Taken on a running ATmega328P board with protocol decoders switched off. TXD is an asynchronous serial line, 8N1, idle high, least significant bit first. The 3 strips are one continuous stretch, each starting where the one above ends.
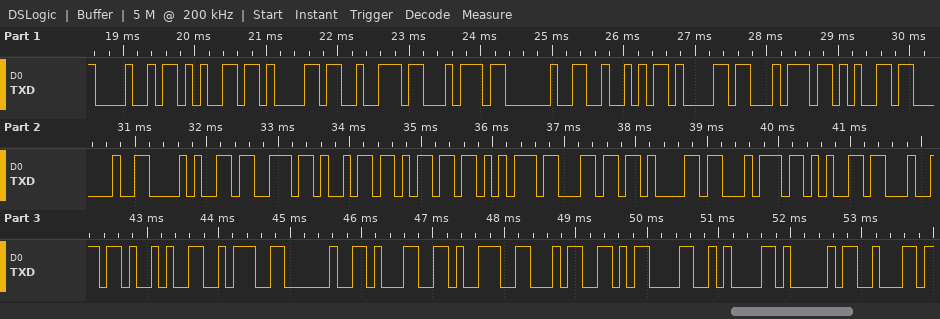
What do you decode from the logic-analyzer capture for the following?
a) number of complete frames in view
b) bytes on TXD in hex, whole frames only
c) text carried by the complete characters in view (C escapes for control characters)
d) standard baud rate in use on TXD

31
0x48 0x65 0x61 0x72 0x74 0x20 0x52 0x61 0x74 0x65 0x20 0x28 0x73 0x69 0x6D 0x75 0x6C 0x61 0x74 0x65 0x64 0x29 0x3A 0x20 0x31 0x39 0x34 0x0D 0x0A 0x41 0x62
"Heart Rate (simulated): 194\r\nAb"
9600 baud
